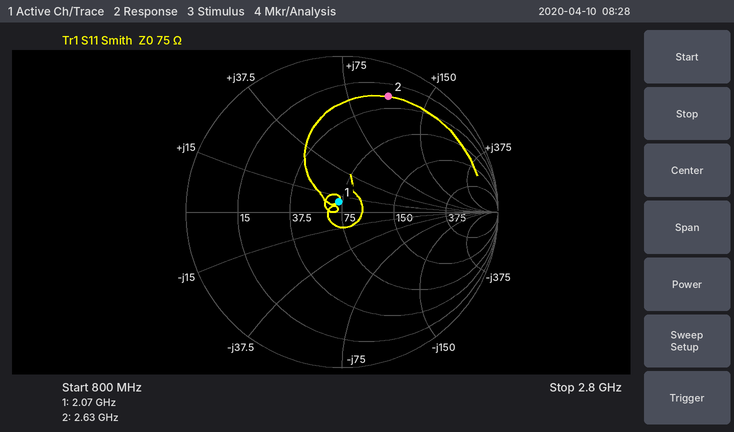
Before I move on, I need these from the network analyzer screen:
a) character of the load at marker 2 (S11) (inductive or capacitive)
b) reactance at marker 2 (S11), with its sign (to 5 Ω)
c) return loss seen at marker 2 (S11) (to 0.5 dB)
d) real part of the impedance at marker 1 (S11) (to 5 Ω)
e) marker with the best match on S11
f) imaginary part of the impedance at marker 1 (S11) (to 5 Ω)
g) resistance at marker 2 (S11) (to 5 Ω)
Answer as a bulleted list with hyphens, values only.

- inductive
- +105 Ω
- 2.0 dB
- 70 Ω
- marker 1
- +10 Ω
- 25 Ω
